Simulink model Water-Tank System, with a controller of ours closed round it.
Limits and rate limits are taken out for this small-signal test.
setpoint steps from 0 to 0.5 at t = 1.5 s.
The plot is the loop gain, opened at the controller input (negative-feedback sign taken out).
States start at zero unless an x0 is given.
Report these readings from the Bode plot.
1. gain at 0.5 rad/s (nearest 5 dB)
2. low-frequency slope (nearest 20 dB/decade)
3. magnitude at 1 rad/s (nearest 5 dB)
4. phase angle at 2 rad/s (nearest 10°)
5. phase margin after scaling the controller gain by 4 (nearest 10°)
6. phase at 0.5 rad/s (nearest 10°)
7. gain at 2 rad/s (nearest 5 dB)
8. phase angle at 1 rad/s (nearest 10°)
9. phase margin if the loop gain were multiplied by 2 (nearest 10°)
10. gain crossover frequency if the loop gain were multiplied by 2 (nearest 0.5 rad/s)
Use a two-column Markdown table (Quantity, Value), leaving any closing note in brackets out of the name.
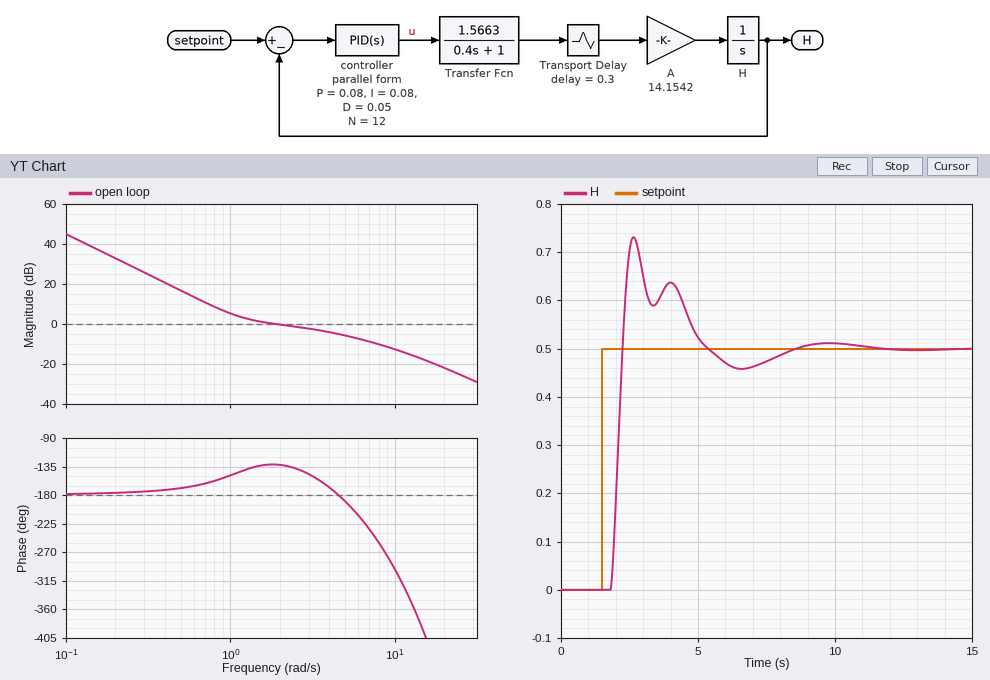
| Quantity | Value |
|---|---|
| gain at 0.5 rad/s | 15 dB |
| low-frequency slope | -40 dB/decade |
| magnitude at 1 rad/s | 5 dB |
| phase angle at 2 rad/s | -130° |
| phase margin after scaling the controller gain by 4 | -110° |
| phase at 0.5 rad/s | -170° |
| gain at 2 rad/s | 0 dB |
| phase angle at 1 rad/s | -150° |
| phase margin if the loop gain were multiplied by 2 | -10° |
| gain crossover frequency if the loop gain were multiplied by 2 | 5.0 rad/s |
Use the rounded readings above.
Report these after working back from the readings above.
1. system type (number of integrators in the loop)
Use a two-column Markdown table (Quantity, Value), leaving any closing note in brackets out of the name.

| Quantity | Value |
|---|---|
| system type | 2 |
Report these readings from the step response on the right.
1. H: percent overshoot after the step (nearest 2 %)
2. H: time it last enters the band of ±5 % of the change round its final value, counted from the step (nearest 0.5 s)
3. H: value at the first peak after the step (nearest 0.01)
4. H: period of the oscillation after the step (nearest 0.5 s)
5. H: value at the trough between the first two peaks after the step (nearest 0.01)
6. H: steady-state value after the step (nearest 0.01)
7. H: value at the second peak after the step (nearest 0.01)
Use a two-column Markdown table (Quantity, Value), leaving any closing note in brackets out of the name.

| Quantity | Value |
|---|---|
| H: percent overshoot after the step | 46 % |
| H: time it last enters the band of ±5 % of the change round its final value, counted from the step | 6.0 s |
| H: value at the first peak after the step | 0.73 |
| H: period of the oscillation after the step | 1.5 s |
| H: value at the trough between the first two peaks after the step | 0.59 |
| H: steady-state value after the step | 0.50 |
| H: value at the second peak after the step | 0.64 |
